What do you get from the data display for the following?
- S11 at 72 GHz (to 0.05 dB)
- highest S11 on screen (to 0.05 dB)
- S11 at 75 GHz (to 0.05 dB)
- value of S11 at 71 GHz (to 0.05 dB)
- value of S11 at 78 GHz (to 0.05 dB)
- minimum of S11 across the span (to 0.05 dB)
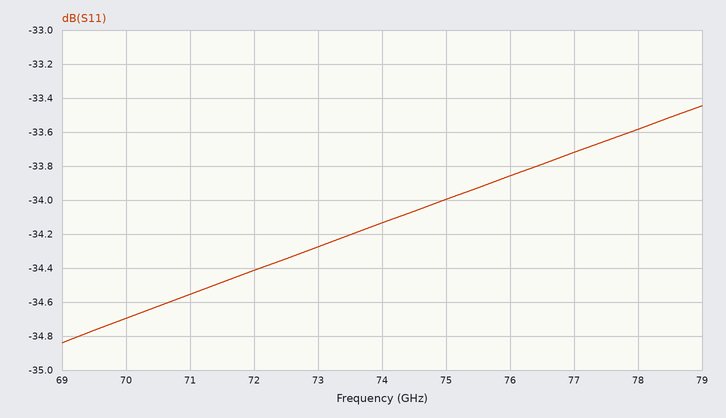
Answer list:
-34.40 dB
-33.45 dB
-34.00 dB
-34.55 dB
-33.60 dB
-34.85 dB
